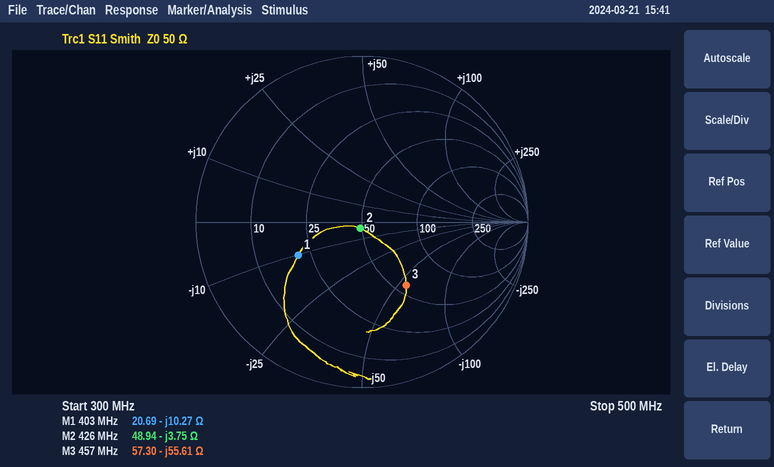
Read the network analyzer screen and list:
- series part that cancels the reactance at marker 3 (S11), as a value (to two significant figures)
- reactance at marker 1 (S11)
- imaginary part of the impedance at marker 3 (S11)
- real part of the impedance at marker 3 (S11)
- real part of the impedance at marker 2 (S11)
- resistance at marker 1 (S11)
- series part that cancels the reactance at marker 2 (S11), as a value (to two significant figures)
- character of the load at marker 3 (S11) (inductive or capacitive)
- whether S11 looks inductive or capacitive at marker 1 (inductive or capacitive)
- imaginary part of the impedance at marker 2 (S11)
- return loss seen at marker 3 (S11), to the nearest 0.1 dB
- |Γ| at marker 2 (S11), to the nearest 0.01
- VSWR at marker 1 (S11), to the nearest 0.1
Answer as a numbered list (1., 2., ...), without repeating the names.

1. 19 nH
2. -10.27 Ω
3. -55.61 Ω
4. 57.30 Ω
5. 48.94 Ω
6. 20.69 Ω
7. 1.4 nH
8. capacitive
9. capacitive
10. -3.75 Ω
11. 6.7 dB
12. 0.04
13. 2.5
